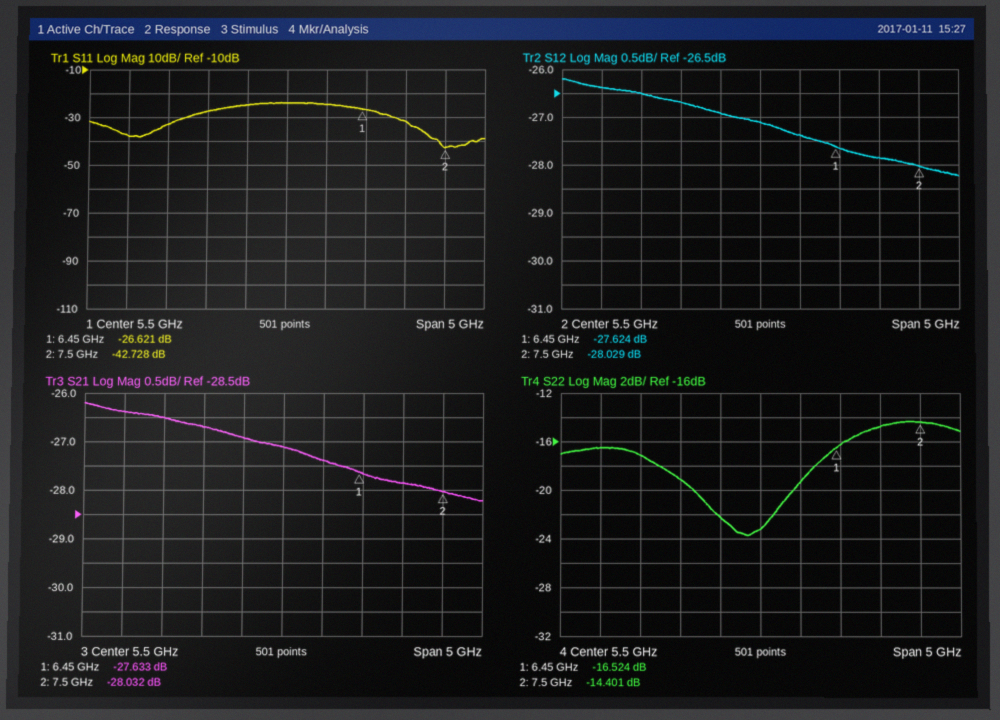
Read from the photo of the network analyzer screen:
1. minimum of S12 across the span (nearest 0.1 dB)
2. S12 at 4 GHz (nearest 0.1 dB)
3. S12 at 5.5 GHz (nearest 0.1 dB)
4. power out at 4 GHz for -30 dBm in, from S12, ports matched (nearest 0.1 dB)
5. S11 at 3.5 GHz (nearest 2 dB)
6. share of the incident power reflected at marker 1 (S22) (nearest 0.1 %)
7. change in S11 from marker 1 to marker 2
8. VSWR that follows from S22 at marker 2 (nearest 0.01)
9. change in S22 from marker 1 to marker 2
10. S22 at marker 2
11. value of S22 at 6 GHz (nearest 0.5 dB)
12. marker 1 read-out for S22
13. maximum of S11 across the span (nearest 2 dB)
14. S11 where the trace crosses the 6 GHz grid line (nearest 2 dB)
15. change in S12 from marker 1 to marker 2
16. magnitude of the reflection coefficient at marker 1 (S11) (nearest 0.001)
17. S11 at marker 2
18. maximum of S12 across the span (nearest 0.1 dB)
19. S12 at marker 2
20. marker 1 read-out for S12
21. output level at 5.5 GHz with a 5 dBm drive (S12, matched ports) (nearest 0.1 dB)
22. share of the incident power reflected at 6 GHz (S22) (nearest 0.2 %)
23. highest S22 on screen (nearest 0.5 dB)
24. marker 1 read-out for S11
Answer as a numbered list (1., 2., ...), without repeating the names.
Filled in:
1. -28.2 dB
2. -26.5 dB
3. -27.1 dB
4. -56.5 dBm
5. -38 dB
6. 2.2 %
7. -16.107 dB
8. 1.47
9. 2.123 dB
10. -14.401 dB
11. -19.5 dB
12. -16.524 dB
13. -24 dB
14. -24 dB
15. -0.405 dB
16. 0.047
17. -42.728 dB
18. -26.2 dB
19. -28.029 dB
20. -27.624 dB
21. -22.1 dBm
22. 1.2 %
23. -14.5 dB
24. -26.621 dB
